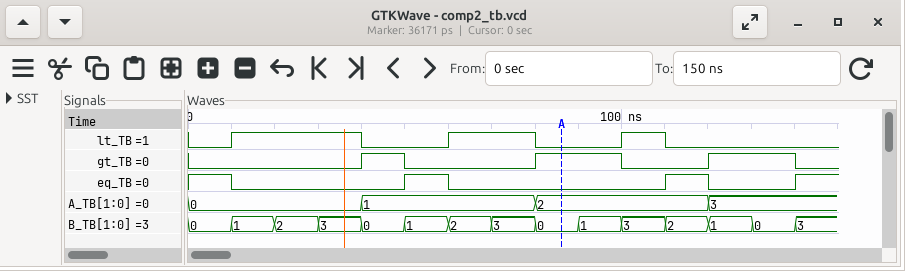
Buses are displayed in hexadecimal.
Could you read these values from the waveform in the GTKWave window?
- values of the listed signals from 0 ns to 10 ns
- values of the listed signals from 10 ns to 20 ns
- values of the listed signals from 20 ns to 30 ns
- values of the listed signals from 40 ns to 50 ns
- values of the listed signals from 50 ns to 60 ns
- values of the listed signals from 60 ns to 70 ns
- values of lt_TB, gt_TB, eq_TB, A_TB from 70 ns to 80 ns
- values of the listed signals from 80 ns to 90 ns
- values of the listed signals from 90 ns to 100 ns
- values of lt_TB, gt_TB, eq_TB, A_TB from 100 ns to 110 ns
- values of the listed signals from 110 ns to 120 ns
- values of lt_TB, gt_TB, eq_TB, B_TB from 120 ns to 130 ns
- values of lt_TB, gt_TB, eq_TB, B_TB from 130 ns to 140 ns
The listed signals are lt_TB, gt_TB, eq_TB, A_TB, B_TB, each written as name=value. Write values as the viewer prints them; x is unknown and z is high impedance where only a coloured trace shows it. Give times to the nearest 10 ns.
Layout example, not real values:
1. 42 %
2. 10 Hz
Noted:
1. lt_TB=0, gt_TB=0, eq_TB=1, A_TB=0, B_TB=0
2. lt_TB=1, gt_TB=0, eq_TB=0, A_TB=0, B_TB=1
3. lt_TB=1, gt_TB=0, eq_TB=0, A_TB=0, B_TB=2
4. lt_TB=0, gt_TB=1, eq_TB=0, A_TB=1, B_TB=0
5. lt_TB=0, gt_TB=0, eq_TB=1, A_TB=1, B_TB=1
6. lt_TB=1, gt_TB=0, eq_TB=0, A_TB=1, B_TB=2
7. lt_TB=1, gt_TB=0, eq_TB=0, A_TB=1
8. lt_TB=0, gt_TB=1, eq_TB=0, A_TB=2, B_TB=0
9. lt_TB=0, gt_TB=1, eq_TB=0, A_TB=2, B_TB=1
10. lt_TB=1, gt_TB=0, eq_TB=0, A_TB=2
11. lt_TB=0, gt_TB=0, eq_TB=1, A_TB=2, B_TB=2
12. lt_TB=0, gt_TB=1, eq_TB=0, B_TB=1
13. lt_TB=0, gt_TB=1, eq_TB=0, B_TB=0
